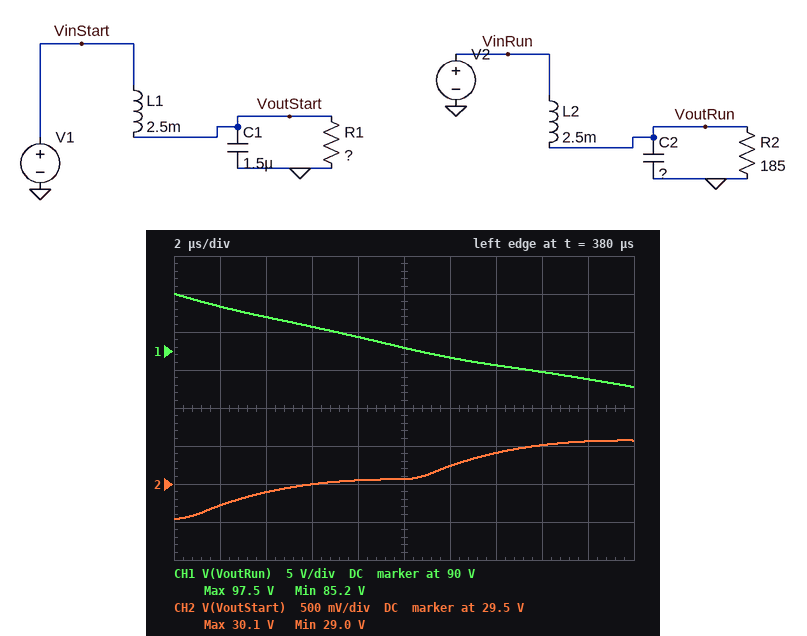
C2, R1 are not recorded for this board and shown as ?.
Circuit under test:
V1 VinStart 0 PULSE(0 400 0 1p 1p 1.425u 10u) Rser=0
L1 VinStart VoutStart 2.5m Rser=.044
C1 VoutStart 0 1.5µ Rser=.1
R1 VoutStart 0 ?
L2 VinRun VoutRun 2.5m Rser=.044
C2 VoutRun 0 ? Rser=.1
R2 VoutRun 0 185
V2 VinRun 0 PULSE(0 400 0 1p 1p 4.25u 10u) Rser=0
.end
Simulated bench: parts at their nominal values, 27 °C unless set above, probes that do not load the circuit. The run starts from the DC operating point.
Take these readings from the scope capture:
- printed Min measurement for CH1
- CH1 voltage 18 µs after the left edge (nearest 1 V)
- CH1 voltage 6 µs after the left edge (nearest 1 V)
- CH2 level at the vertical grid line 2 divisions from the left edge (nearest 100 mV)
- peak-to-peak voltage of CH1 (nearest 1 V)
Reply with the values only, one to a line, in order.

85.2 V
86 V
93 V
29.4 V
12 V
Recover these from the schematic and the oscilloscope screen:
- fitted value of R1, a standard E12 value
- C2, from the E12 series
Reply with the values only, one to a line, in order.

4.7 Ω
1.8 µF
